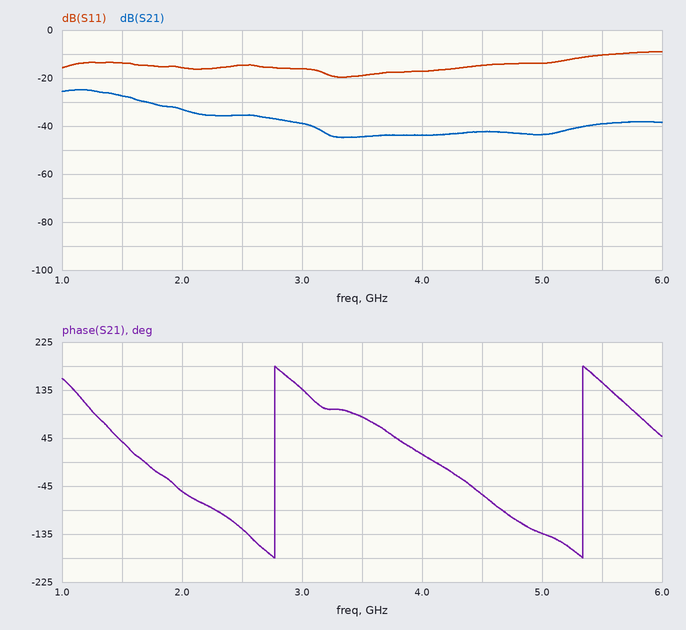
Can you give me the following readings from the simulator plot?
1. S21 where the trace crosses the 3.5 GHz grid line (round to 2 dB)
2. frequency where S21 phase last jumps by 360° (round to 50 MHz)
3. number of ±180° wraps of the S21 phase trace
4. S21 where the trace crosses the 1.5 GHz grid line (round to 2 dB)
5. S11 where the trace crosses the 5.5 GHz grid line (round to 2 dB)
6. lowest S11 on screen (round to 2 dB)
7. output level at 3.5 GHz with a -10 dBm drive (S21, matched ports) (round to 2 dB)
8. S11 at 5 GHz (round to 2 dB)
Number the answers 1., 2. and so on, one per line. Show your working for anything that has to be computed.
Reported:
1. -44 dB
2. 5.35 GHz
3. 2
4. -28 dB
5. -10 dB
6. -20 dB
7. -10 dBm + (-44 dB) = -54 dBm
8. -14 dB
